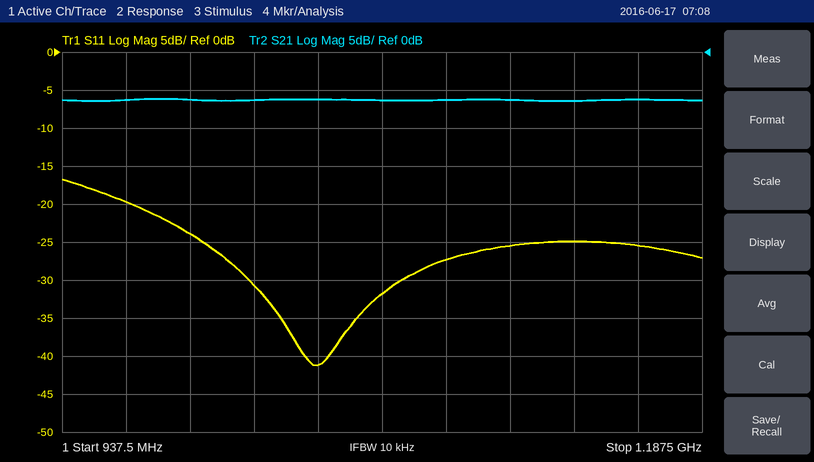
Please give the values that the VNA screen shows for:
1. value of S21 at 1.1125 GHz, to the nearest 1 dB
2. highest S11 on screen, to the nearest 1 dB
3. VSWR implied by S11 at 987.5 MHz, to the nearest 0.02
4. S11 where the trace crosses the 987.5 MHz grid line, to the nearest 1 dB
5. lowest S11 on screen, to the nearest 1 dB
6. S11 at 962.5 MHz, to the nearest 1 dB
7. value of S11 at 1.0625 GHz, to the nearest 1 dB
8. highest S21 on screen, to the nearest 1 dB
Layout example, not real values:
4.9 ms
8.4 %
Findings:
-6 dB
-17 dB
1.14
-24 dB
-41 dB
-20 dB
-32 dB
-6 dB
